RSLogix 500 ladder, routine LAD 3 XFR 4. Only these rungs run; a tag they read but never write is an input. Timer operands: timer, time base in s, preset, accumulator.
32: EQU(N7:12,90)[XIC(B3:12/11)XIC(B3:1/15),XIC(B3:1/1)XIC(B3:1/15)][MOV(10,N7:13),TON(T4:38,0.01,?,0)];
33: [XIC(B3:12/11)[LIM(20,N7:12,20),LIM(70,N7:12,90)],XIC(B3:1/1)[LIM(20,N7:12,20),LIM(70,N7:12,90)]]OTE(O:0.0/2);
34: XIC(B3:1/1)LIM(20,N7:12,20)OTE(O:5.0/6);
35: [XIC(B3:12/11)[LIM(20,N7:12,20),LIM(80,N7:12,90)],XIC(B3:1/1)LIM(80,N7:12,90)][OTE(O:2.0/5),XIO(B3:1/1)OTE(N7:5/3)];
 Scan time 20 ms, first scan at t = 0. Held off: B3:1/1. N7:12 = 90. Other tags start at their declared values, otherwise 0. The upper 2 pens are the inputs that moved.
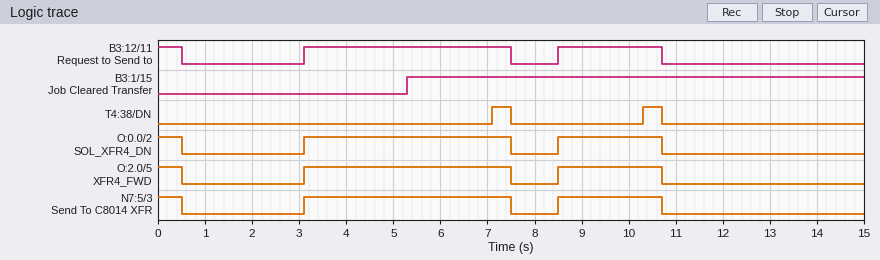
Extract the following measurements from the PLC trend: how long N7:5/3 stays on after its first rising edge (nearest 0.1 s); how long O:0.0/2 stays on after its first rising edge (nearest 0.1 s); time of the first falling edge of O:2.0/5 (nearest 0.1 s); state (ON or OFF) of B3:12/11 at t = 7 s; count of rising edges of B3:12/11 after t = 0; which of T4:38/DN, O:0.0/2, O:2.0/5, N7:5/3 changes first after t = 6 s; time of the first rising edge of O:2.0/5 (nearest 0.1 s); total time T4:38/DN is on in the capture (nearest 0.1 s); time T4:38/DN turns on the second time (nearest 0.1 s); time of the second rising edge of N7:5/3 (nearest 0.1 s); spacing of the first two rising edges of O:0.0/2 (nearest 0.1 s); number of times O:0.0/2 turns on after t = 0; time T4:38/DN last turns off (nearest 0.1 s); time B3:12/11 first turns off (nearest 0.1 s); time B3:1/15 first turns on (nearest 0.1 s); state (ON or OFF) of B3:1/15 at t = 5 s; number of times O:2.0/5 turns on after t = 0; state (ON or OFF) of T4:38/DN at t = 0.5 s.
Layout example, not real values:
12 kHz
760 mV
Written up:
4.4 s
4.4 s
0.5 s
ON
2
T4:38/DN
3.1 s
0.8 s
10.3 s
8.5 s
5.4 s
2
10.7 s
0.5 s
5.3 s
OFF
2
OFF
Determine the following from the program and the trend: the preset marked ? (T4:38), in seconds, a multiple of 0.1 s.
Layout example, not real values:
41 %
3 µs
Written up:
1.8 s
